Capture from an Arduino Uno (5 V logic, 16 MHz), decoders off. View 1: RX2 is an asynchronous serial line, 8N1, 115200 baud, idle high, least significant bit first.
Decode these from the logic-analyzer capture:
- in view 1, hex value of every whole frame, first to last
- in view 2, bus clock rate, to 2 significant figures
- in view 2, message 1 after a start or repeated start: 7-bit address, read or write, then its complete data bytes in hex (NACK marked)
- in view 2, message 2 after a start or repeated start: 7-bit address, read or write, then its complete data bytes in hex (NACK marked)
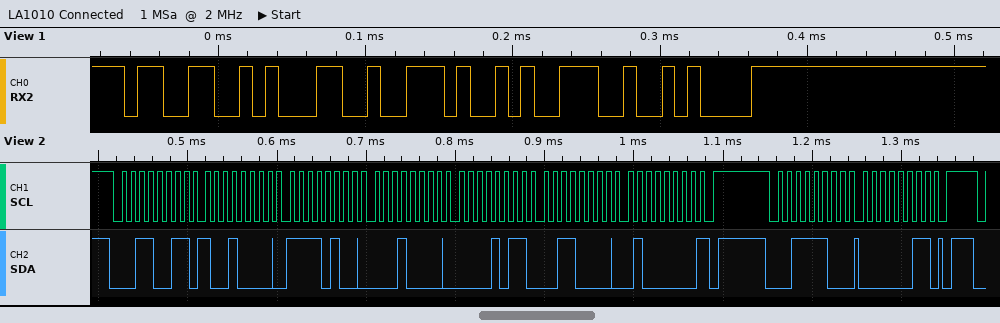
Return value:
33 31 2E 39 0A
100 kHz
0x19 read: 90 F4 10 0B 30 40 NACK
0x1E write: 03
